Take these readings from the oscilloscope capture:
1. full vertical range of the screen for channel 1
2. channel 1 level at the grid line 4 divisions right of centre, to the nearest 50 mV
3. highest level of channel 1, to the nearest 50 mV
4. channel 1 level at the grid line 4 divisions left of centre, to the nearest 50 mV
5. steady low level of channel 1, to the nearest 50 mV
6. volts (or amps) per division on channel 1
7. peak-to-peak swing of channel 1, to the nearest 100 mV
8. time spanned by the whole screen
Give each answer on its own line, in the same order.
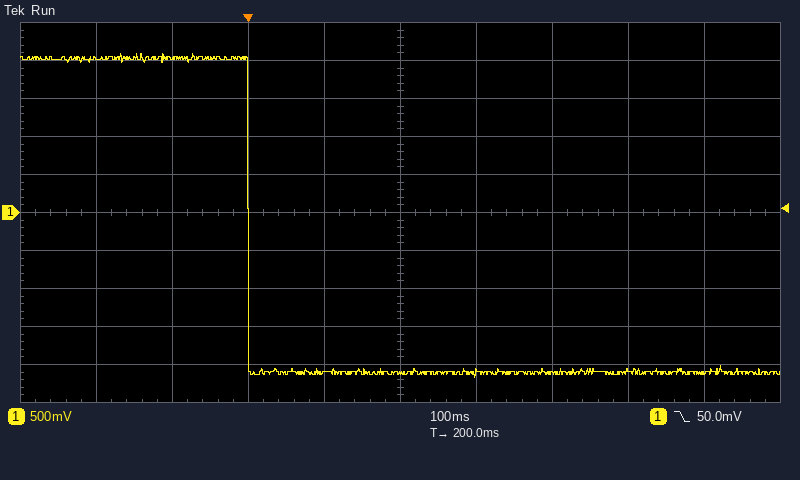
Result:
5 V
-2.10 V
2.10 V
2.05 V
-2.10 V
500 mV
4.30 V
1 s
